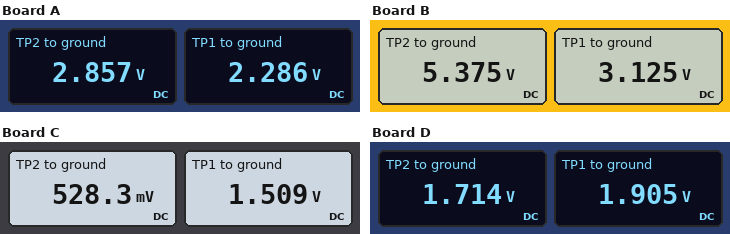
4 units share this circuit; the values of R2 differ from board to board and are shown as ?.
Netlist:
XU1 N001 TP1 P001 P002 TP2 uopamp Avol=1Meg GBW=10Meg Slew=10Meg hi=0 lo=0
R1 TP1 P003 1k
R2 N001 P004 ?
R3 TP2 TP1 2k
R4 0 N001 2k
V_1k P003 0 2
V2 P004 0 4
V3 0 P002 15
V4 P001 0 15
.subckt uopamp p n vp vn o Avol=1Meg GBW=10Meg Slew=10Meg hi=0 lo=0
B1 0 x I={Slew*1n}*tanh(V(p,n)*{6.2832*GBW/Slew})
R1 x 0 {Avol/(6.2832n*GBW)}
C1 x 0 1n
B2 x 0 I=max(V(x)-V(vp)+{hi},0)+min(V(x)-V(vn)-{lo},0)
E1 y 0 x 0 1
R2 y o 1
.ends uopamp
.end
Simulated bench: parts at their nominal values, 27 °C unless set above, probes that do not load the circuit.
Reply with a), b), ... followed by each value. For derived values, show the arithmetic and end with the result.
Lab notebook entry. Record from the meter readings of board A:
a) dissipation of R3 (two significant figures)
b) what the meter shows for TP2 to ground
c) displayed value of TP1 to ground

a) (2.857 V - 2.286 V)^2 / 2 kΩ = 160 µW
b) 2.857 V
c) 2.286 V
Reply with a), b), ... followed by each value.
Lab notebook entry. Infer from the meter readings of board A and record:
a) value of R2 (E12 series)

a) 1.5 kΩ
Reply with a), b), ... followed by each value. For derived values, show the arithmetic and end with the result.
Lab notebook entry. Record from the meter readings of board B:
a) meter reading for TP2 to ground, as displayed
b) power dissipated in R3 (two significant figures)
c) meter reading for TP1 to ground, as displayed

a) 5.375 V
b) (5.375 V - 3.125 V)^2 / 2 kΩ = 2.5 mW
c) 3.125 V
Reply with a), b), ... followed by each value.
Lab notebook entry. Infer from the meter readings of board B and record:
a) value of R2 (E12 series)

a) 560 Ω
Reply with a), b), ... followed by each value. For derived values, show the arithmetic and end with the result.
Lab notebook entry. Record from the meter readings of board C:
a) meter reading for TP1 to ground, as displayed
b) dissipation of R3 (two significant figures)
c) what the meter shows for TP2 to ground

a) 1.509 V
b) (1.509 V - 528.3 mV)^2 / 2 kΩ = 480 µW
c) 528.3 mV
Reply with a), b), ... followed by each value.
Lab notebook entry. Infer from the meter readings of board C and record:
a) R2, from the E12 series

a) 3.3 kΩ
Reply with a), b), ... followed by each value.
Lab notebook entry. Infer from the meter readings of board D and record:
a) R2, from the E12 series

a) 2.2 kΩ
